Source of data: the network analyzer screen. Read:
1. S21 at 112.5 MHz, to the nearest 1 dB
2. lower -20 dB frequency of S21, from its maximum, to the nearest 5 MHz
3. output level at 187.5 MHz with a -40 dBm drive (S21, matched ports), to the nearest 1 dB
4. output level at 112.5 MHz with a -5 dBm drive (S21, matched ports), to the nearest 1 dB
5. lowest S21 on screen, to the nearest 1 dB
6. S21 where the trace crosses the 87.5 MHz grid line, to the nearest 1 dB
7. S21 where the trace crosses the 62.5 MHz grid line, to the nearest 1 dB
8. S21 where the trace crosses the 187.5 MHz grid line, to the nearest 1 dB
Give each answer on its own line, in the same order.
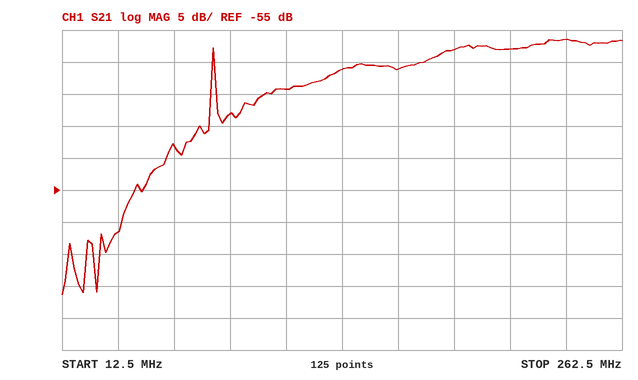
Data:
-39 dB
55 MHz
-73 dBm
-44 dBm
-71 dB
-43 dB
-48 dB
-33 dB
